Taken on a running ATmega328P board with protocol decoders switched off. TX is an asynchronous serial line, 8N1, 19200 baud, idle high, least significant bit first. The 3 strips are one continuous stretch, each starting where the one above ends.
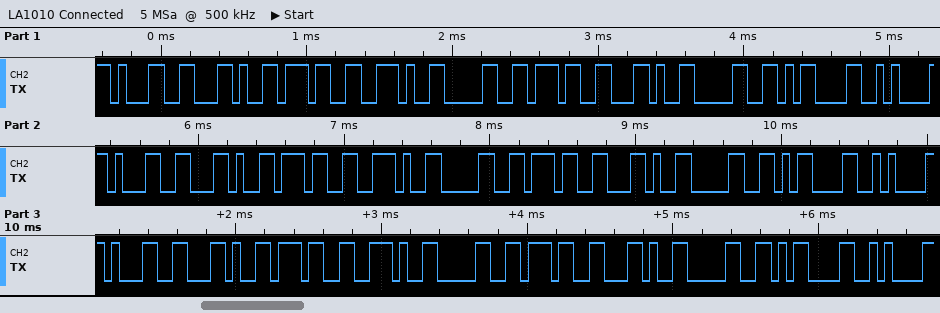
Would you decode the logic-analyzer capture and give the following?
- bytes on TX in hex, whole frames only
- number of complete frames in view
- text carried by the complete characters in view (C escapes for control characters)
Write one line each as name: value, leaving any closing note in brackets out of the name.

bytes on TX in hex, whole frames only: 31 2C 37 2E 30 37 2C 30 0D 0A 31 2C 37 2E 30 37 2C 30 0D 0A 31 2C 37 2E 30 37 2C 30 0D 0A
number of complete frames in view: 30
text carried by the complete characters in view: "1,7.07,0\r\n1,7.07,0\r\n1,7.07,0\r\n"
